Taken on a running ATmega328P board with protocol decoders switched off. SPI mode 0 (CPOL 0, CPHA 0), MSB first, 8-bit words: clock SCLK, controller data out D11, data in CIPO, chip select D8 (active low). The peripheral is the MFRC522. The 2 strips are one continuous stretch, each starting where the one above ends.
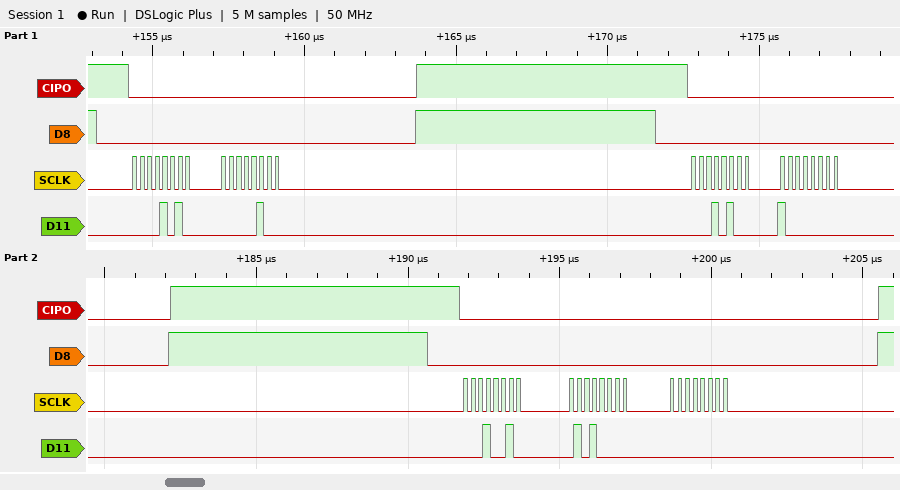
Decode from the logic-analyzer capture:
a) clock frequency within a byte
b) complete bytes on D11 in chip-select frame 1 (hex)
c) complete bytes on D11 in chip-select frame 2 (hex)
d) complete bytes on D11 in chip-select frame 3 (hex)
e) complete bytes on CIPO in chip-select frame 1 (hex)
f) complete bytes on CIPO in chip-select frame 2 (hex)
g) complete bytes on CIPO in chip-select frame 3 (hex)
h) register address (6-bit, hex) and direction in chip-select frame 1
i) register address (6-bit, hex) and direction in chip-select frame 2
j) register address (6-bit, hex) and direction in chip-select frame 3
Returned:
4 MHz
0x0A 0x04
0x14 0x80
0x12 0x50 0x00
0x00 0x00
0x00 0x00
0x00 0x00 0x00
0x05 write
0x0A write
0x09 write
